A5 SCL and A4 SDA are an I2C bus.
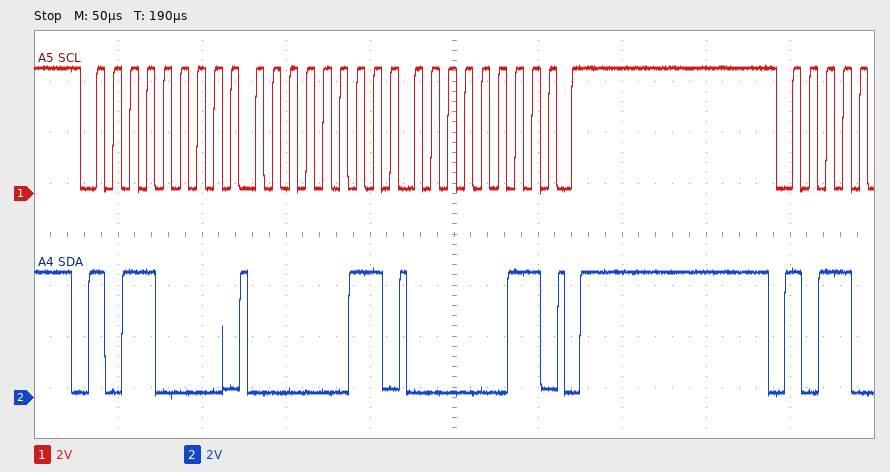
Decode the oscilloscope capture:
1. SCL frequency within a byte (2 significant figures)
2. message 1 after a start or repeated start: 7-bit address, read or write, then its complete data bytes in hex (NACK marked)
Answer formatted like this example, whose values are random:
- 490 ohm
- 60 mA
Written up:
- 100 kHz
- 0x58 write: 03 03
